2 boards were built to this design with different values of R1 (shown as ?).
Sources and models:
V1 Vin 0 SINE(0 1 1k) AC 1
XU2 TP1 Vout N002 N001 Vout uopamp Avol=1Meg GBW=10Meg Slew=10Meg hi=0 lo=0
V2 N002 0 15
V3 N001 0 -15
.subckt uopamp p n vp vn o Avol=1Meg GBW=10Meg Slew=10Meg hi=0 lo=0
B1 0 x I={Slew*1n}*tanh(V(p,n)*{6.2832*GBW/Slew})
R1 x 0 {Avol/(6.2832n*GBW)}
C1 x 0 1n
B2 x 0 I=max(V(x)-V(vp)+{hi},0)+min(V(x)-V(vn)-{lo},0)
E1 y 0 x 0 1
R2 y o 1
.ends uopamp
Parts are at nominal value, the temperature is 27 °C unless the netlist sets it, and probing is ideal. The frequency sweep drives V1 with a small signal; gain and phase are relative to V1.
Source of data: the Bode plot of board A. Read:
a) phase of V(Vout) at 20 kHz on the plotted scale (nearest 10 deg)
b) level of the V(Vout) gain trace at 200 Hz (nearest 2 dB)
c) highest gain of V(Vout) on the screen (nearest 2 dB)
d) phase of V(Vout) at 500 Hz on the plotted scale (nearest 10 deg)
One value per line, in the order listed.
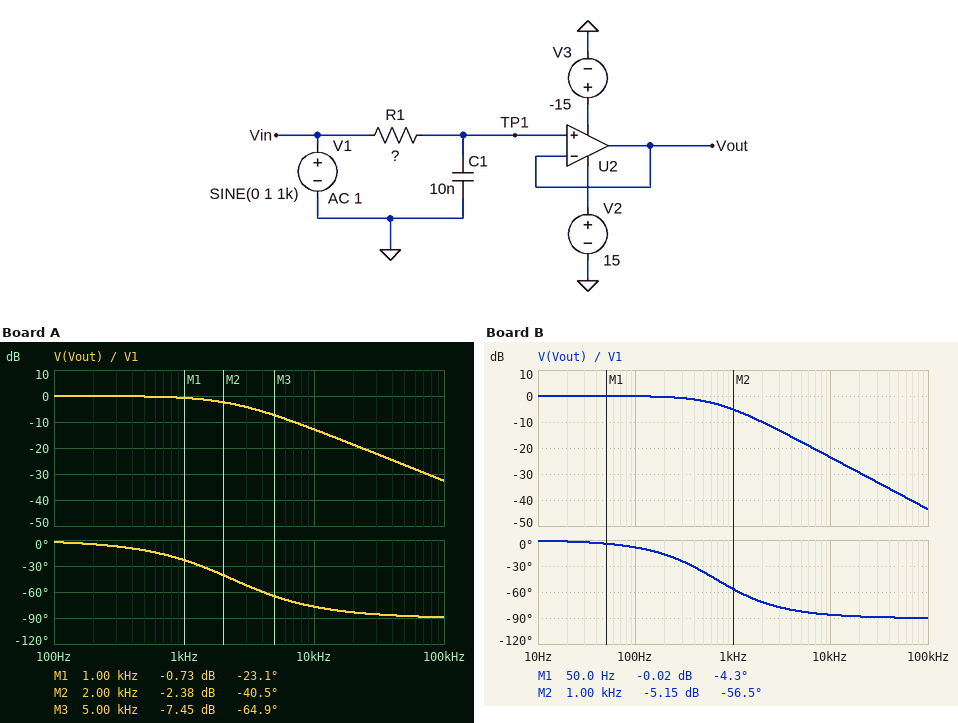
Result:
-80 deg
0 dB
0 dB
-10 deg
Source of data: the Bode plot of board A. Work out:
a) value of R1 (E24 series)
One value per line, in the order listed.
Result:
6.8 kΩ
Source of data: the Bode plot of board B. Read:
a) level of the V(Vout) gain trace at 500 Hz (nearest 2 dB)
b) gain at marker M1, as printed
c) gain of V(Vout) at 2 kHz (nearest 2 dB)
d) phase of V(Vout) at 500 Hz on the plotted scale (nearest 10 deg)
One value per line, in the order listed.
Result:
-2 dB
-0.02 dB
-10 dB
-40 deg
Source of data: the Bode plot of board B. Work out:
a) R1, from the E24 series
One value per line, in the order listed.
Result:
24 kΩ
